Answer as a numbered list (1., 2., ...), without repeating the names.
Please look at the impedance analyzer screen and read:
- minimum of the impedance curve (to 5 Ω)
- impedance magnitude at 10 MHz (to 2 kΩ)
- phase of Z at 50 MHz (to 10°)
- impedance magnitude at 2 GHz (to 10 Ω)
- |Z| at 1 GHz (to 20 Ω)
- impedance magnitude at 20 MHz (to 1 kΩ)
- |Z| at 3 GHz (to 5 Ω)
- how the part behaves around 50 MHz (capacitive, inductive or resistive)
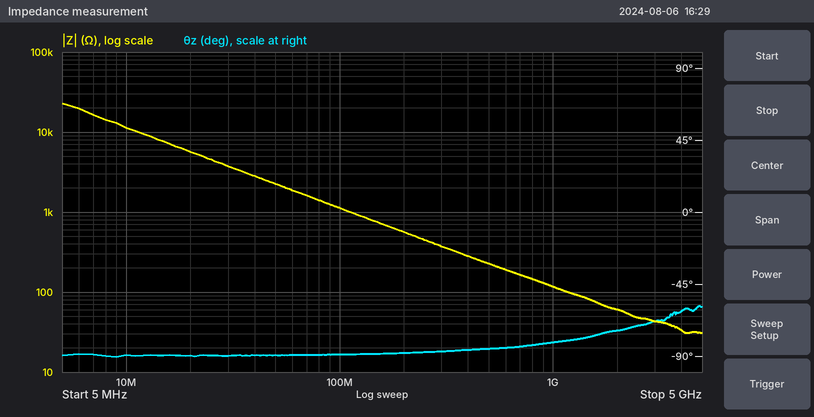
1. 30 Ω
2. 12 kΩ
3. -90°
4. 60 Ω
5. 120 Ω
6. 6 kΩ
7. 45 Ω
8. capacitive
